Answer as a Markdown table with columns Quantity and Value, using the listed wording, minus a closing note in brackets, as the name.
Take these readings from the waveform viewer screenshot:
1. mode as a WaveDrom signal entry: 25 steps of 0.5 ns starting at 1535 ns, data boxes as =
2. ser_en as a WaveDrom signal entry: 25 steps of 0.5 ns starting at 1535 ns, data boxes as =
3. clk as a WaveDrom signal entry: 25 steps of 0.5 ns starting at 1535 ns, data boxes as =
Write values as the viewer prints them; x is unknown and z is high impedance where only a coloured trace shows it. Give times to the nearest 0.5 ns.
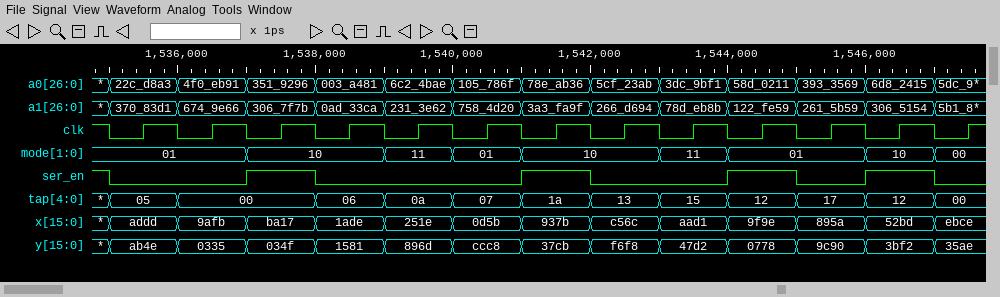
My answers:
| Quantity | Value |
|---|---|
| mode as a WaveDrom signal entry: 25 steps of 0.5 ns starting at 1535 ns, data boxes as = | {name: 'mode', wave: '=...=...=.=.=...=.=...=.=', data: '01 10 11 01 10 11 01 10 00'} |
| ser_en as a WaveDrom signal entry: 25 steps of 0.5 ns starting at 1535 ns, data boxes as = | {name: 'ser_en', wave: '0...1.0.....1.0...1.0.1.0'} |
| clk as a WaveDrom signal entry: 25 steps of 0.5 ns starting at 1535 ns, data boxes as = | {name: 'clk', wave: '0101010101010101010101010'} |
